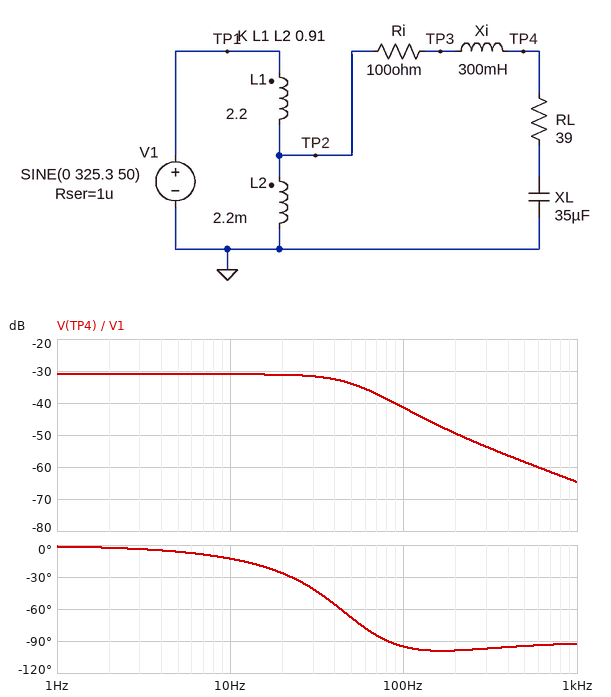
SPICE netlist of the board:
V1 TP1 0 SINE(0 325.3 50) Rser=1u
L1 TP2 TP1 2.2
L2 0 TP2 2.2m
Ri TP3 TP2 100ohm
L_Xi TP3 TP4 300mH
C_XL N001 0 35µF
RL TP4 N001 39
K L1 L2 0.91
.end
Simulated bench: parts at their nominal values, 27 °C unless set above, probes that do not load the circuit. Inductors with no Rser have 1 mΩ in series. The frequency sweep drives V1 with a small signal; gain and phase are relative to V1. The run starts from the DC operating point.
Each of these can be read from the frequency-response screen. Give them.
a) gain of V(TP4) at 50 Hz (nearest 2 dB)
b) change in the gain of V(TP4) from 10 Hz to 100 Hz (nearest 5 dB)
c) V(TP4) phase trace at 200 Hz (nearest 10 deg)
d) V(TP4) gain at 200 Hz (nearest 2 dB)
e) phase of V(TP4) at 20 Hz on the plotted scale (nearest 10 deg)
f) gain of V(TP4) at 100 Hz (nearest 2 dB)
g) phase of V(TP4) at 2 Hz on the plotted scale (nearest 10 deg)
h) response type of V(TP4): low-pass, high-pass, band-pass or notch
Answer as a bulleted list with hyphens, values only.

- -34 dB
- -10 dB
- -100 deg
- -50 dB
- -30 deg
- -42 dB
- 0 deg
- low-pass
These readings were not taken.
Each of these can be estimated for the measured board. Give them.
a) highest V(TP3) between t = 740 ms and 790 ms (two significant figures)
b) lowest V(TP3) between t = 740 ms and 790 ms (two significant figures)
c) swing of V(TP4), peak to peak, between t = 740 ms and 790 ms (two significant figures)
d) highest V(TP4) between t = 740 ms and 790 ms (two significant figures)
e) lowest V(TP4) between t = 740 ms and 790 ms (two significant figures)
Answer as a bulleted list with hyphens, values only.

- 2.6 V
- -2.6 V
- 13 V
- 6.5 V
- -6.5 V
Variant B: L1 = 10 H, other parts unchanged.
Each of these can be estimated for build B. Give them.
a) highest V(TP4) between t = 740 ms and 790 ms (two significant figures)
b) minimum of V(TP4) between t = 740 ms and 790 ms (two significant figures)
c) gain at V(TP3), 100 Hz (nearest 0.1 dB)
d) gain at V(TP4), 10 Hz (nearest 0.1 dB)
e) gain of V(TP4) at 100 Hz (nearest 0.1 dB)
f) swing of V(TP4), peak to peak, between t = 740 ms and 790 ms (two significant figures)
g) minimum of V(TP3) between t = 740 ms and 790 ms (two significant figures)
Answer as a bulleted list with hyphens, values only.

- 3.1 V
- -3.1 V
- -40.1 dB
- -37.5 dB
- -47.9 dB
- 6.2 V
- -1.2 V
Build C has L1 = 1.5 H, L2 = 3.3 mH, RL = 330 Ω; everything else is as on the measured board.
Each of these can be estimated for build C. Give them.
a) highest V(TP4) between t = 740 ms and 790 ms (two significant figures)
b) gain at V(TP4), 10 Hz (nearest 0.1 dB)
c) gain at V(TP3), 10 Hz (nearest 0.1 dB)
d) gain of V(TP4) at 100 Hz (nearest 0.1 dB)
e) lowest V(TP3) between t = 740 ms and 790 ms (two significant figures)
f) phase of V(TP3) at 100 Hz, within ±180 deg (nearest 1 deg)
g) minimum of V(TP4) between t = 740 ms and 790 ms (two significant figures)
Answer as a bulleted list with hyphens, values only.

- 11 V
- -28.4 dB
- -28.7 dB
- -30.4 dB
- -10 V
- 5 deg
- -11 V
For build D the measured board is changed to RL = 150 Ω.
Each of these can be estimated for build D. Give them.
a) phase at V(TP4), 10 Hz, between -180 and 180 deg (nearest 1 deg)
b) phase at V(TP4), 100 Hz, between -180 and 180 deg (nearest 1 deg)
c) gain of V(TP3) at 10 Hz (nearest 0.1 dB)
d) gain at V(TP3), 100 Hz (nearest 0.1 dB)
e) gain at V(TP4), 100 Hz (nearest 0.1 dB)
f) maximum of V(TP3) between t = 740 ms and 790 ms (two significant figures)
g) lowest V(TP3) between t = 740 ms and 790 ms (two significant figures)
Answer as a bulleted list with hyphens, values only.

- -12 deg
- -47 deg
- -31.8 dB
- -33.9 dB
- -36.3 dB
- 5.5 V
- -5.5 V
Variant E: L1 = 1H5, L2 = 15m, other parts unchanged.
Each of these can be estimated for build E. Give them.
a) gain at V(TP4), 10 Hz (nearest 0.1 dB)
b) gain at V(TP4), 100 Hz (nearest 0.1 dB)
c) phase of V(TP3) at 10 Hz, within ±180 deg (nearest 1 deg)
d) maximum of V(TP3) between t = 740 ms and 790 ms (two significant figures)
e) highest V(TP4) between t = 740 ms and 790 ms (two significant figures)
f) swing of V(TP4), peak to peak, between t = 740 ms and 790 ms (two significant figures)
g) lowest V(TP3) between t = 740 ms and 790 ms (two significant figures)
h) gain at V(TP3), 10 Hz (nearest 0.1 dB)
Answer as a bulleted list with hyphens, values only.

- -21.5 dB
- -31.9 dB
- -13 deg
- 7.8 V
- 20 V
- 39 V
- -7.8 V
- -21.8 dB
